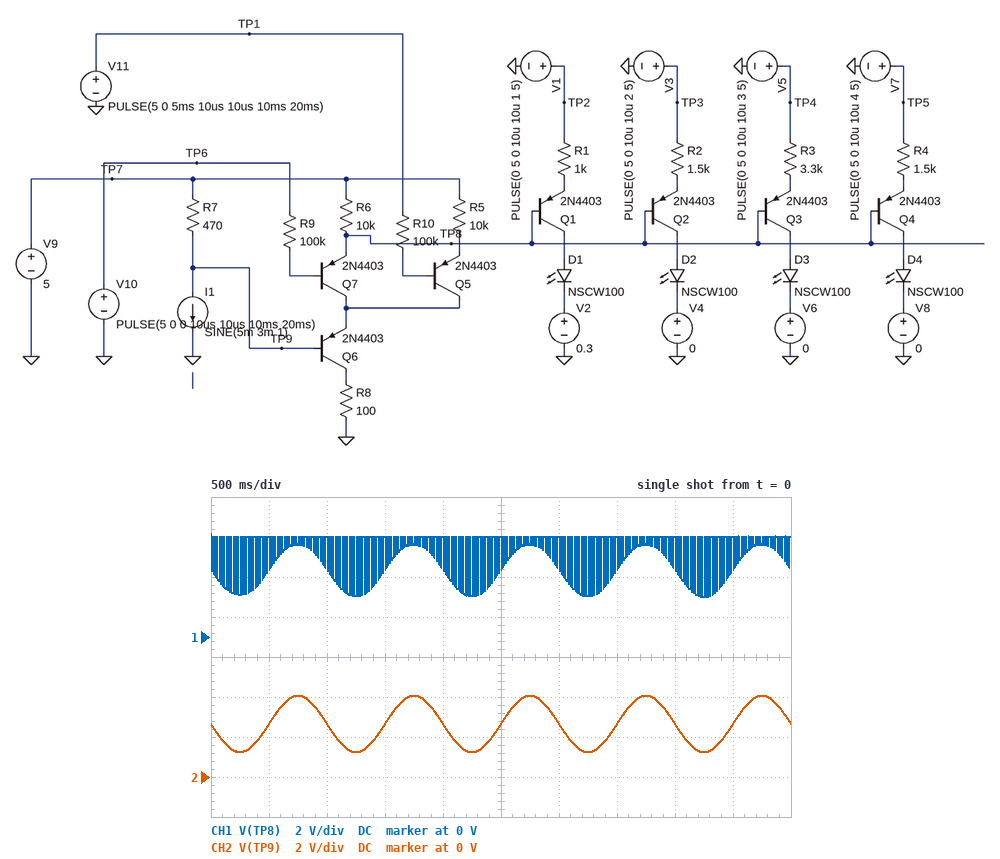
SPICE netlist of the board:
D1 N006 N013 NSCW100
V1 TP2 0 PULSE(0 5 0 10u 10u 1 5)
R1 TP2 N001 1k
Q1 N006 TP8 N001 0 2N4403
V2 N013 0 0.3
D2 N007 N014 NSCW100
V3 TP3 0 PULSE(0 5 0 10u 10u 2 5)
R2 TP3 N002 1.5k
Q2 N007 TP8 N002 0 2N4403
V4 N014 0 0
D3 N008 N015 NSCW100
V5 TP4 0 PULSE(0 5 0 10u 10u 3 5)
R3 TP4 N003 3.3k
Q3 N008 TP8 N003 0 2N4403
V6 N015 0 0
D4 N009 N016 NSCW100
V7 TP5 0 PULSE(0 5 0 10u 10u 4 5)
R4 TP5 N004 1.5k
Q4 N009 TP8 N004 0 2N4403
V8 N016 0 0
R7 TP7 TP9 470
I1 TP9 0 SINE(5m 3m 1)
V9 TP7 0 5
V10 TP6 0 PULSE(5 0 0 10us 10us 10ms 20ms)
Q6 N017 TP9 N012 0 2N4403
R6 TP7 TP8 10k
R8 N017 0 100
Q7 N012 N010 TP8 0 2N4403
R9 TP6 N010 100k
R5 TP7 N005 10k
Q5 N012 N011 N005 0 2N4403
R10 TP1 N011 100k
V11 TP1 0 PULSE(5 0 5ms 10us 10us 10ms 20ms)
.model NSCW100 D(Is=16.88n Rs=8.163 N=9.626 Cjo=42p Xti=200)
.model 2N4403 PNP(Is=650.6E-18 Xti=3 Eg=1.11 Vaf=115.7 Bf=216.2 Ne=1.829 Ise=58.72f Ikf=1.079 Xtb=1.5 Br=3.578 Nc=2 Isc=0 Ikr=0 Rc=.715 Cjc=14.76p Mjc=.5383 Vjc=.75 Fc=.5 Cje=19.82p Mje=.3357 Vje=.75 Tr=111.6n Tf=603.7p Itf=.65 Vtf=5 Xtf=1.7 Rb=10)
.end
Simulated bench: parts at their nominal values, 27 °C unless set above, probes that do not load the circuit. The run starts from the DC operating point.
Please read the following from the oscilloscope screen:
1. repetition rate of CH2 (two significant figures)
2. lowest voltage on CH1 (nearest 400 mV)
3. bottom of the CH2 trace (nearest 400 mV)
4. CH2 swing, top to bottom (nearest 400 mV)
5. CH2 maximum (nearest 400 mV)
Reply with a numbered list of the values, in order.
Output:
1. 1.0 Hz
2. 2.0 V
3. 1.2 V
4. 2.8 V
5. 4.0 V
